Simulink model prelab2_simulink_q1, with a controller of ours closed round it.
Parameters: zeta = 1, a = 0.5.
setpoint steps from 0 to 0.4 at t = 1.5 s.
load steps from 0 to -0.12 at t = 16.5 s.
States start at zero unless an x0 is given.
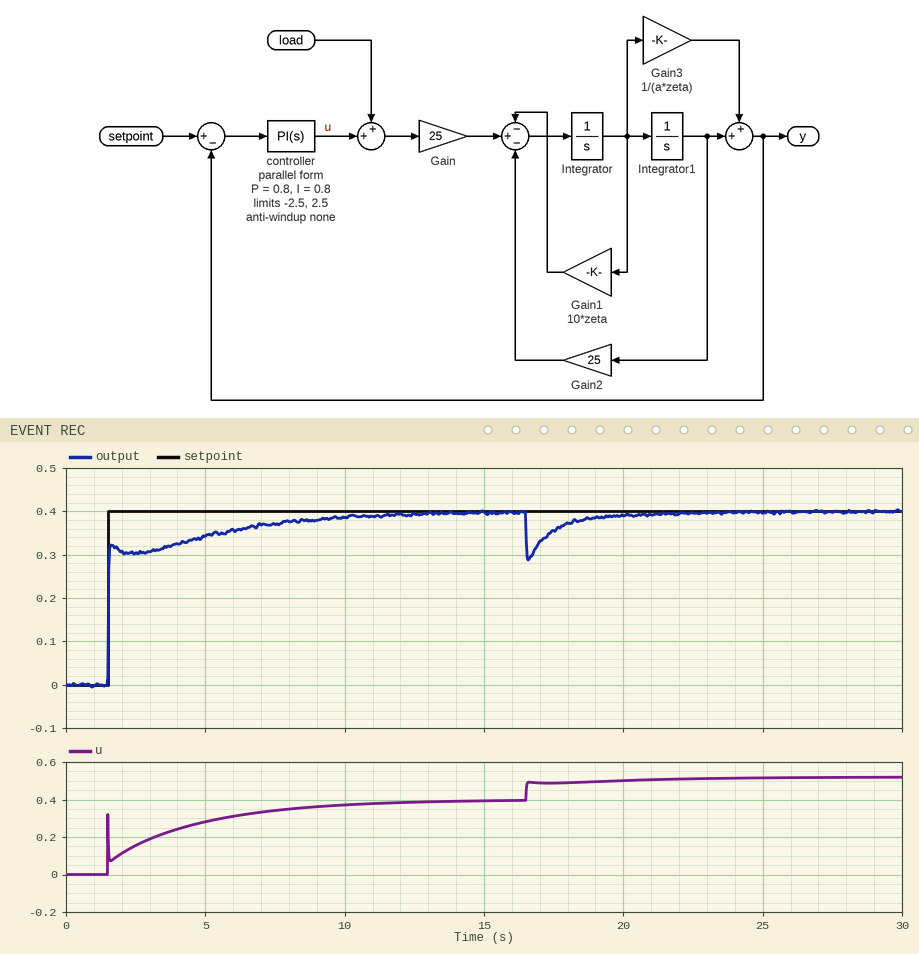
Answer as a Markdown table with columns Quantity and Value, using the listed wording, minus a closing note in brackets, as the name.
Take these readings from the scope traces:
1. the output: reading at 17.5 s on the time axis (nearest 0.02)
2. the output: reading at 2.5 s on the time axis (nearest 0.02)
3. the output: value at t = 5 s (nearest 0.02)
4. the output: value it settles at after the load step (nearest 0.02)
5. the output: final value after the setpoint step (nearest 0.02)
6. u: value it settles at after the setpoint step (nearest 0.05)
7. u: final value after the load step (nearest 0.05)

| Quantity | Value |
|---|---|
| the output: reading at 17.5 s on the time axis | 0.36 |
| the output: reading at 2.5 s on the time axis | 0.30 |
| the output: value at t = 5 s | 0.34 |
| the output: value it settles at after the load step | 0.40 |
| the output: final value after the setpoint step | 0.40 |
| u: value it settles at after the setpoint step | 0.40 |
| u: final value after the load step | 0.50 |
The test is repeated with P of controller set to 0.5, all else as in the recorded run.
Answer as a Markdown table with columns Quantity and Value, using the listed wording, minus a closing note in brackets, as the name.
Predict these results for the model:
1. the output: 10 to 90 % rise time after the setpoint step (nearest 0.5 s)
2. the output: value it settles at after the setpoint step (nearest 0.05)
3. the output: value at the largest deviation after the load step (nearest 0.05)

| Quantity | Value |
|---|---|
| the output: 10 to 90 % rise time after the setpoint step | 4.5 s |
| the output: value it settles at after the setpoint step | 0.40 |
| the output: value at the largest deviation after the load step | 0.25 |
